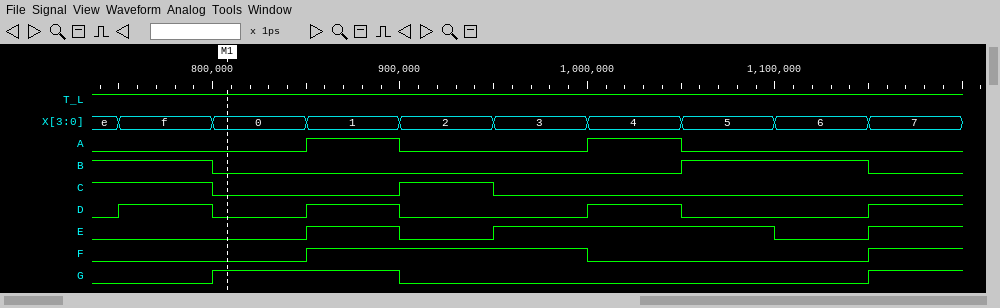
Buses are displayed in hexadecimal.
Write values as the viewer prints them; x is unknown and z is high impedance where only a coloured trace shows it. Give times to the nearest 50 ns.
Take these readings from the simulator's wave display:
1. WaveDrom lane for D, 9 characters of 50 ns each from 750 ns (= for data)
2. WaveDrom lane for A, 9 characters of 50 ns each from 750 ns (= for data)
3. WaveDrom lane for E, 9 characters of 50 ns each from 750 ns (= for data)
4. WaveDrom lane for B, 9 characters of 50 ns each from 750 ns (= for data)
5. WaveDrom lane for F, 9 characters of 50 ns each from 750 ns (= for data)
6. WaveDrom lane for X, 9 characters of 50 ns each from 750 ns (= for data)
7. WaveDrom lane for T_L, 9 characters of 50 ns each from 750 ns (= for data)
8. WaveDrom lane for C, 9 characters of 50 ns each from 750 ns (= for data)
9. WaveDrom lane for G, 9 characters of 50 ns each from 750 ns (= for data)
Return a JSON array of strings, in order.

["{name: 'D', wave: '1010.10.1'}", "{name: 'A', wave: '0.10.10..'}", "{name: 'E', wave: '0.101..01'}", "{name: 'B', wave: '10....1.0'}", "{name: 'F', wave: '0.1..0..1'}", "{name: 'X', wave: '=========', data: 'f 0 1 2 3 4 5 6 7'}", "{name: 'T_L', wave: '1........'}", "{name: 'C', wave: '10.10....'}", "{name: 'G', wave: '01.0....1'}"]
